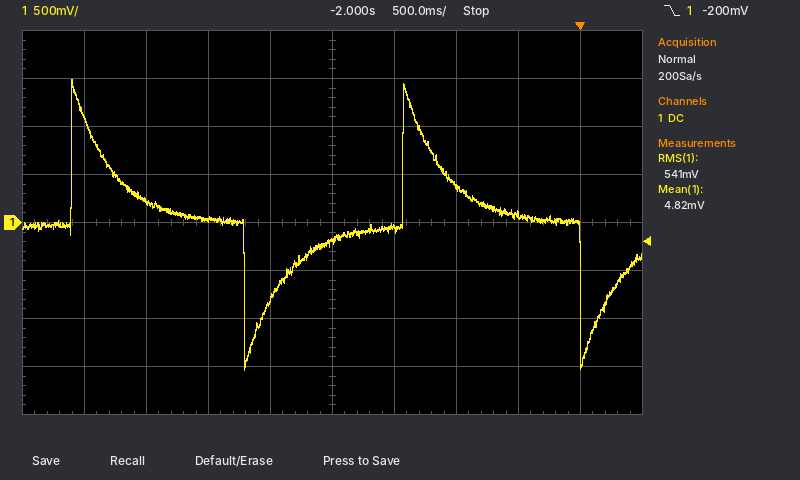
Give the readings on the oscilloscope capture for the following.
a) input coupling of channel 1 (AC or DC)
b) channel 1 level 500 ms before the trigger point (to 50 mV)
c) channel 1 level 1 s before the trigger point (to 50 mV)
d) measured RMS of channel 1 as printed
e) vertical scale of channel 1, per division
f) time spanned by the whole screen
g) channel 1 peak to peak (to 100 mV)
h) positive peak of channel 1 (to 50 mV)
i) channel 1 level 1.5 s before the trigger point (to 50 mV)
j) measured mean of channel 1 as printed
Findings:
DC
100 mV
400 mV
541 mV
500 mV
5 s
3.00 V
1.50 V
-50 mV
4.82 mV
